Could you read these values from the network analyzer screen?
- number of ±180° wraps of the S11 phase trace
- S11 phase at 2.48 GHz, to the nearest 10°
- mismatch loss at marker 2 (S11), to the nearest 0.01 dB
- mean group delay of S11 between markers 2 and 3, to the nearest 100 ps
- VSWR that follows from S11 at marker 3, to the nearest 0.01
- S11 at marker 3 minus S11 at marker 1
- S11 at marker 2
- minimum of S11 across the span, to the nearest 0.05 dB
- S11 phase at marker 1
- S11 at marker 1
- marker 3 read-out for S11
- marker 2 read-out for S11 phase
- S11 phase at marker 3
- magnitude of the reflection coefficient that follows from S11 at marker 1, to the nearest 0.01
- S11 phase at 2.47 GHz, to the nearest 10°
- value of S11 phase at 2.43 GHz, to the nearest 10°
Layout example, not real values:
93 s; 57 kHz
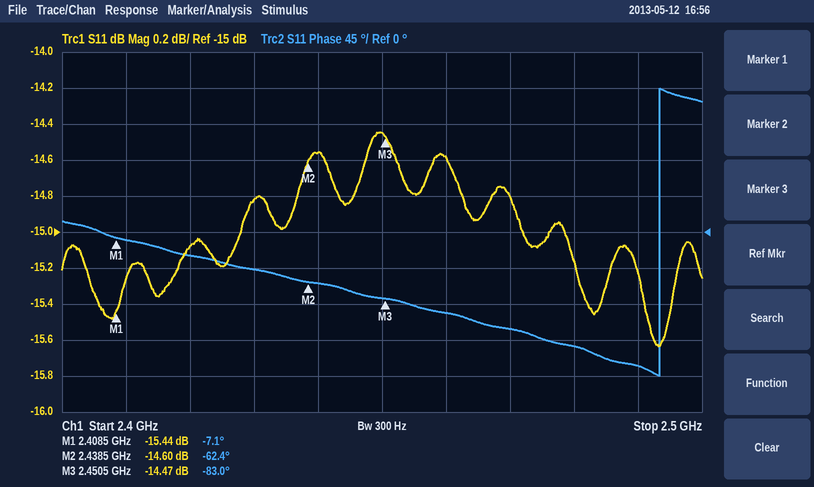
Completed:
1; -140°; 0.15 dB; 4.8 ns; 1.47; 0.97 dB; -14.60 dB; -15.65 dB; -7.1°; -15.44 dB; -14.47 dB; -62.4°; -83.0°; 0.17; -120°; -50°
